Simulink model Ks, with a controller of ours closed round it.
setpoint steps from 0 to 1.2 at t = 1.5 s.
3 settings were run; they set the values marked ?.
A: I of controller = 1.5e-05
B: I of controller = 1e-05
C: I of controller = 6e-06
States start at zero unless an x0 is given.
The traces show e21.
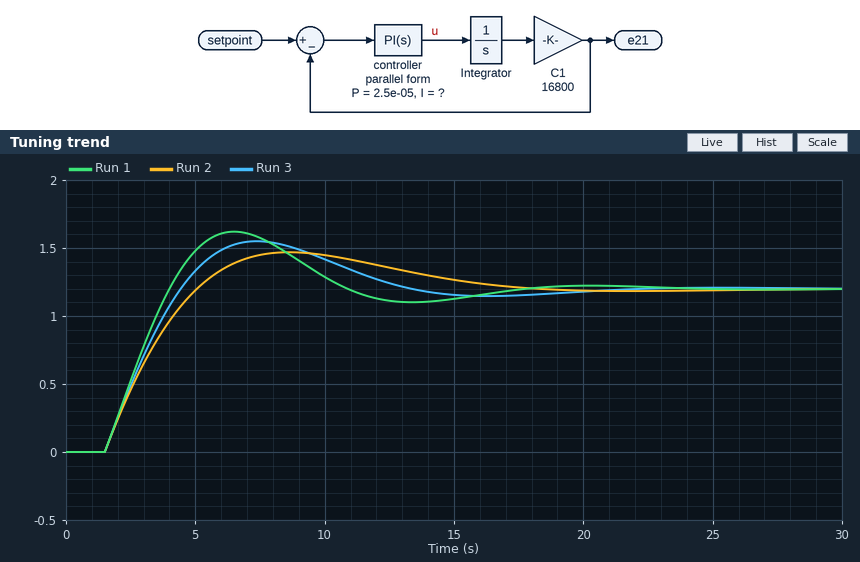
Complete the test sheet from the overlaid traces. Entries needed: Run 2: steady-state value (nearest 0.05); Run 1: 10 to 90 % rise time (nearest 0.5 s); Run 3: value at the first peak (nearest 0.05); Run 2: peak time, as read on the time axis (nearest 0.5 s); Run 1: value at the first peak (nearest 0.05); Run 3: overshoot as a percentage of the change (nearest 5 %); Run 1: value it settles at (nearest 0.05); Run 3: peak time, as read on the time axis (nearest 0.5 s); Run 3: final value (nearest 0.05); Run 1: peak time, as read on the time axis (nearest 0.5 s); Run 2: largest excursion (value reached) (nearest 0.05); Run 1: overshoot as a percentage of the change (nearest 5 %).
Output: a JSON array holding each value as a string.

["1.20", "2.0 s", "1.55", "8.5 s", "1.60", "30 %", "1.20", "7.5 s", "1.20", "6.5 s", "1.45", "35 %"]
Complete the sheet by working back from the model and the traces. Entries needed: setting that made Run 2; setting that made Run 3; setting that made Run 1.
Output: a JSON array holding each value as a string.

["C", "B", "A"]
